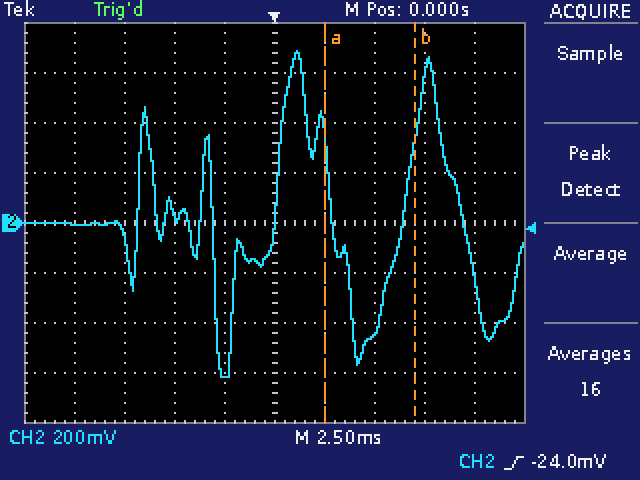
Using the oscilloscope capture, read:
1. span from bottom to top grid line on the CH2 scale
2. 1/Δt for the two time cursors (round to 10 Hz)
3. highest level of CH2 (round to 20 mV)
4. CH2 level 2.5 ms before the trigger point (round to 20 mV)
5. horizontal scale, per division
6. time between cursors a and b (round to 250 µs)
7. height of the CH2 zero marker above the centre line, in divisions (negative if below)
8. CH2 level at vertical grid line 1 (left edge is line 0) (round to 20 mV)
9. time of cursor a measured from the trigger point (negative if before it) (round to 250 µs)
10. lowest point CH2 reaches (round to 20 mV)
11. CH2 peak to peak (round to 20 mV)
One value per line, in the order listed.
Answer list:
1.6 V
220 Hz
680 mV
-600 mV
2.5 ms
4.50 ms
0.0 div
0 mV
+2.50 ms
-620 mV
1.30 V
